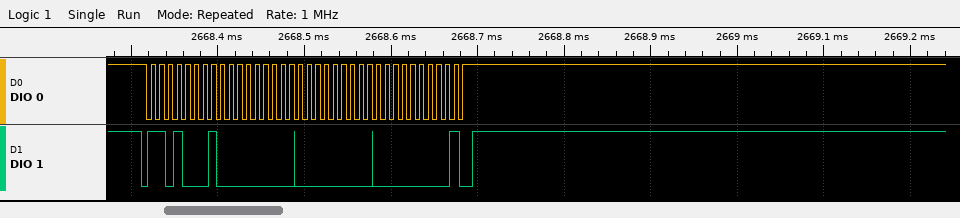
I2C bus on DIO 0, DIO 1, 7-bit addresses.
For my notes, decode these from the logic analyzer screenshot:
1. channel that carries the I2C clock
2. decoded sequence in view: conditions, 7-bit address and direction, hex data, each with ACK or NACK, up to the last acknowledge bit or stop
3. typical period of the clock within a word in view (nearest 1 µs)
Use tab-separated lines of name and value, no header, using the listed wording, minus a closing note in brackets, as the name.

channel that carries the I2C clock	DIO 0
decoded sequence in view: conditions, 7-bit address and direction, hex data, each with ACK or NACK, up to the last acknowledge bit or stop	start, address 68 read ACK, 00 ACK, 00 ACK, 00 NACK, stop
typical period of the clock within a word in view	10 µs
